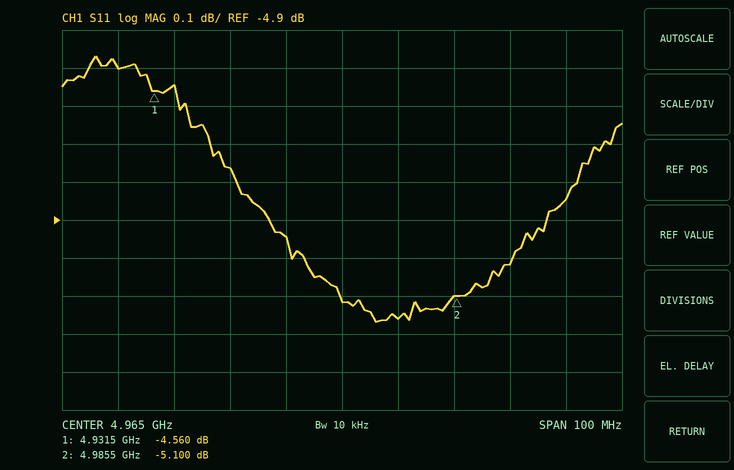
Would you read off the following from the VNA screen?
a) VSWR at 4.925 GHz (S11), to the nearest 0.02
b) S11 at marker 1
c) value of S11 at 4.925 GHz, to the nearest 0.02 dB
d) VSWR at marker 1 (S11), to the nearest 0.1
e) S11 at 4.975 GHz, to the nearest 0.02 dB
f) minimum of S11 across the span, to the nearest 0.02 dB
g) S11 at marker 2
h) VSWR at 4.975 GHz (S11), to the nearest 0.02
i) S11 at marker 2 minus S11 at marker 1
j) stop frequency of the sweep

3.94
-4.560 dB
-4.50 dB
3.9
-5.16 dB
-5.16 dB
-5.100 dB
3.46
-0.540 dB
5.015 GHz
